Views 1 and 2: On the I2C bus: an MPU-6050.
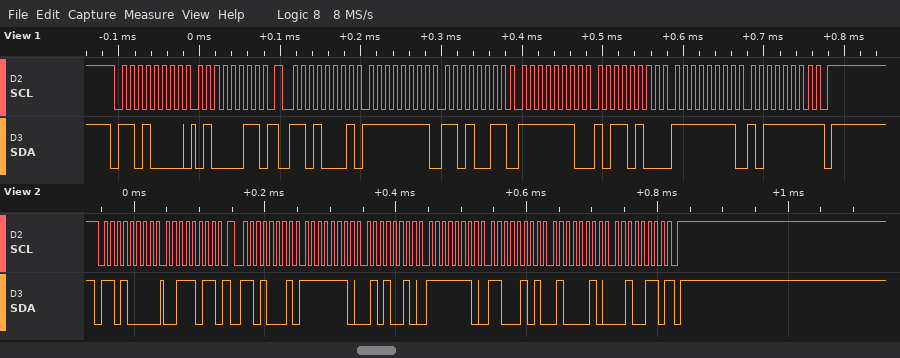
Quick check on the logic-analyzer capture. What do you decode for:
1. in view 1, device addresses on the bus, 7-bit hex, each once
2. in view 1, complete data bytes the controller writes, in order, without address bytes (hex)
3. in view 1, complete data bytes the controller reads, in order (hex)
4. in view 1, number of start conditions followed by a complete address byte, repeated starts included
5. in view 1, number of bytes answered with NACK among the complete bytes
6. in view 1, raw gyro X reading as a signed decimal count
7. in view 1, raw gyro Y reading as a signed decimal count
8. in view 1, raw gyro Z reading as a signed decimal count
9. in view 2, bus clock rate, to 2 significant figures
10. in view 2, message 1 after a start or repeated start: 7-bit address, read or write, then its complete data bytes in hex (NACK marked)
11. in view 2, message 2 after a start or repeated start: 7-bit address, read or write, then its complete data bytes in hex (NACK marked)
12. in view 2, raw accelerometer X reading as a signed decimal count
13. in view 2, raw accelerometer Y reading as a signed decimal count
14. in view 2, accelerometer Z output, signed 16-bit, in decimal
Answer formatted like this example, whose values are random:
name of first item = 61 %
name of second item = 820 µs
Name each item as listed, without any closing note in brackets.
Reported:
in view 1, device addresses on the bus, 7-bit hex, each once = 0x68
in view 1, complete data bytes the controller writes, in order, without address bytes = 43
in view 1, complete data bytes the controller reads, in order = FF D3 FE B4 FF BF
in view 1, number of start conditions followed by a complete address byte, repeated starts included = 2
in view 1, number of bytes answered with NACK among the complete bytes = 1
in view 1, raw gyro X reading as a signed decimal count = -45
in view 1, raw gyro Y reading as a signed decimal count = -332
in view 1, raw gyro Z reading as a signed decimal count = -65
in view 2, bus clock rate, to 2 significant figures = 100 kHz
in view 2, message 1 after a start or repeated start: 7-bit address, read or write, then its complete data bytes in hex = 0x68 write: 3B
in view 2, message 2 after a start or repeated start: 7-bit address, read or write, then its complete data bytes in hex = 0x68 read: FE 52 FE C5 42 26 NACK
in view 2, raw accelerometer X reading as a signed decimal count = -430
in view 2, raw accelerometer Y reading as a signed decimal count = -315
in view 2, accelerometer Z output, signed 16-bit, in decimal = 16934
